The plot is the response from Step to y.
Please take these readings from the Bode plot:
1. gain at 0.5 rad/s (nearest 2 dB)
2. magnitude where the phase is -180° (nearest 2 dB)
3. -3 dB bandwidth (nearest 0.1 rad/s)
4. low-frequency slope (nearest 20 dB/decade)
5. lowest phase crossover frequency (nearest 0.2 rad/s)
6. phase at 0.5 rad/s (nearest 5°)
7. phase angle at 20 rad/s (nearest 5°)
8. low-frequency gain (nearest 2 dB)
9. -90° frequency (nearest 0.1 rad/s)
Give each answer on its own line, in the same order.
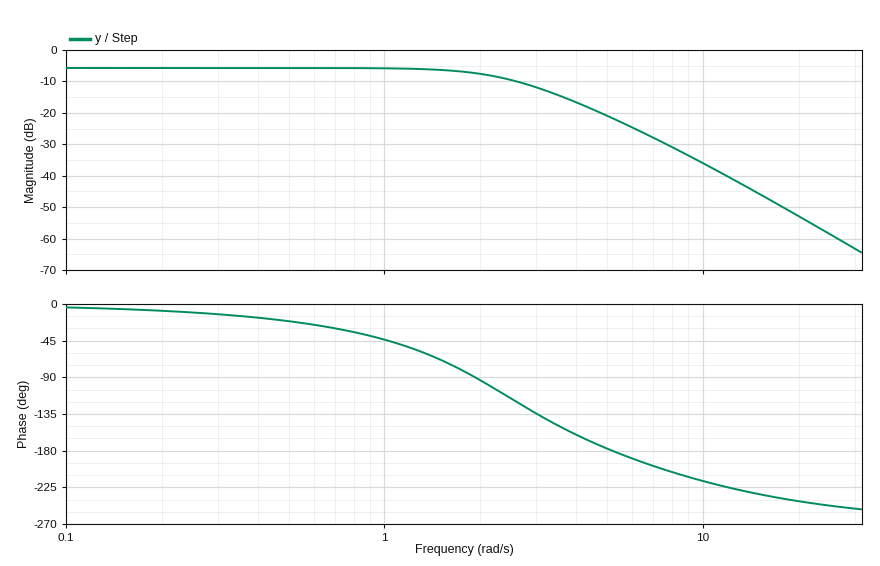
-6 dB
-22 dB
2.3 rad/s
0 dB/decade
5.2 rad/s
-20°
-240°
-6 dB
1.9 rad/s
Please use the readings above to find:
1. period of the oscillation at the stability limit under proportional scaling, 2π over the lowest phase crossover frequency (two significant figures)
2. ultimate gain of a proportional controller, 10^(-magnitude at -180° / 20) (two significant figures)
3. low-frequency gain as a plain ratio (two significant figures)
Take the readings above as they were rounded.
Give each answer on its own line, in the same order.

1.2 s
13
0.50
